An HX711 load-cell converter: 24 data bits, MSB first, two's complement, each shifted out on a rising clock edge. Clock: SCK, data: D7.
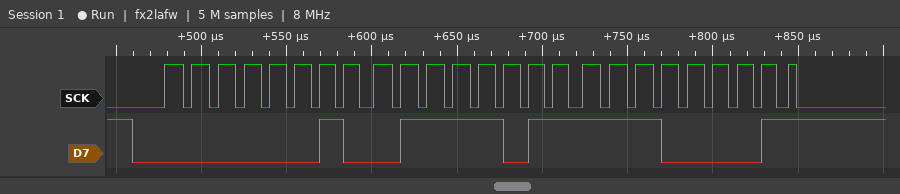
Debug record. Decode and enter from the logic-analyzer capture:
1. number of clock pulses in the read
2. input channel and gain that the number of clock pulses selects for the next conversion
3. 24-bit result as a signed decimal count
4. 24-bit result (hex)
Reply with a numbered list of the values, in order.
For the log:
1. 25
2. channel A, gain 128
3. 162785
4. 0x027BE1
